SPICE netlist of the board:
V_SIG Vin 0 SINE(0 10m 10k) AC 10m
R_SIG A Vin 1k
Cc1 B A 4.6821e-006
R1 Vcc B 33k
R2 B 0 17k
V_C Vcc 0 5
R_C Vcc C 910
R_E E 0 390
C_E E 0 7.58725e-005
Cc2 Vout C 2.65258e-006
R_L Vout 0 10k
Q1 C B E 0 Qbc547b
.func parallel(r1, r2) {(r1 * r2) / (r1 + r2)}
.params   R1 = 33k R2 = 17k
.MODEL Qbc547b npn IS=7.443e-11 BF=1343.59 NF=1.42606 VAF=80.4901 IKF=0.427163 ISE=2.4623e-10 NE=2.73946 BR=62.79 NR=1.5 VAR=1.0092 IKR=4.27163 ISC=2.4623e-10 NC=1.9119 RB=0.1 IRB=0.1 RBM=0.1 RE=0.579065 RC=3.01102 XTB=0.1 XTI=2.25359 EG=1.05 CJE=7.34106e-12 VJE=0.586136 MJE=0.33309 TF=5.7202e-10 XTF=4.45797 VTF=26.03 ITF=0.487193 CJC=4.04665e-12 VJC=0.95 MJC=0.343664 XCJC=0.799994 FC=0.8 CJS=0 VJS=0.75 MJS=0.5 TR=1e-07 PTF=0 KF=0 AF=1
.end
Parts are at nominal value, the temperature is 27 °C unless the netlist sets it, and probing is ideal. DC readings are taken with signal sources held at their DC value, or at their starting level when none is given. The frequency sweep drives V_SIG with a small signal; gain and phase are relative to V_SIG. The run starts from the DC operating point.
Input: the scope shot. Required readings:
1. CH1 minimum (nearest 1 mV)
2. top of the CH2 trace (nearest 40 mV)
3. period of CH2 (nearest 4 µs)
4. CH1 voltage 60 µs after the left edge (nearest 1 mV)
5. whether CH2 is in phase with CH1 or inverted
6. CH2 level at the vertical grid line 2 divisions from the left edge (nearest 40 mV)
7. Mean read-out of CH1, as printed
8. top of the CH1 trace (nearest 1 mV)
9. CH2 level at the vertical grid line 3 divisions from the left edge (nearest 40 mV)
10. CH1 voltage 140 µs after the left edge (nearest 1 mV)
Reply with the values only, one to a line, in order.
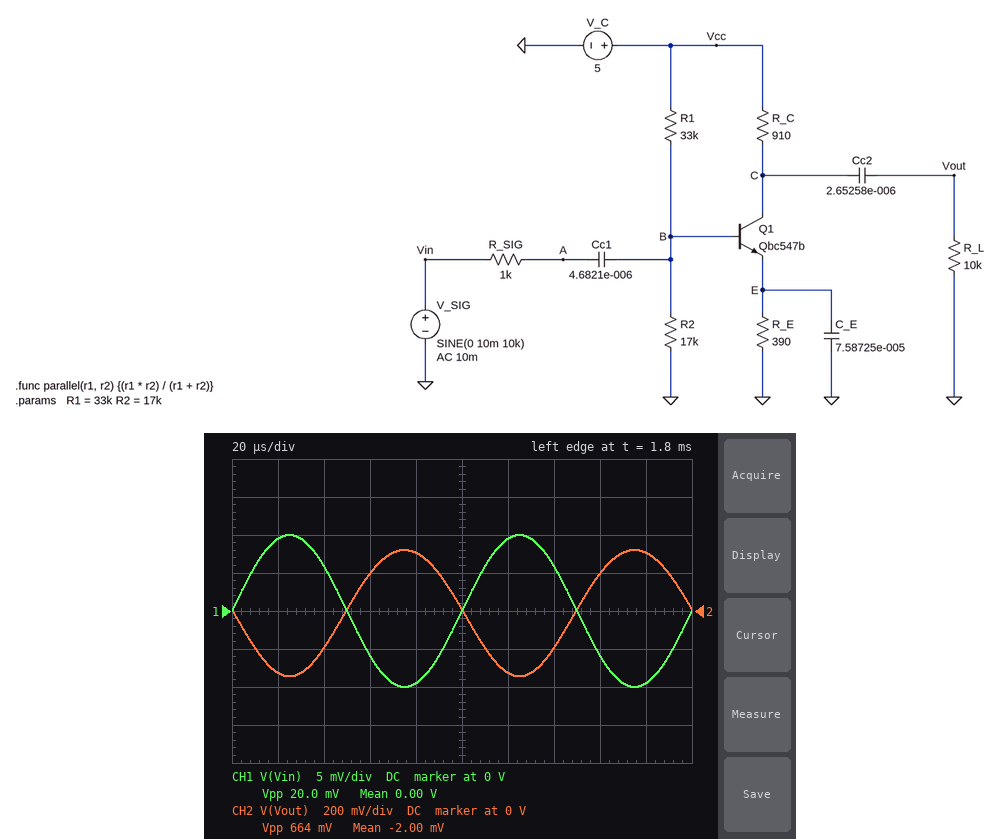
-10 mV
320 mV
100 µs
-6 mV
inverted
-200 mV
0.00 V
10 mV
200 mV
6 mV
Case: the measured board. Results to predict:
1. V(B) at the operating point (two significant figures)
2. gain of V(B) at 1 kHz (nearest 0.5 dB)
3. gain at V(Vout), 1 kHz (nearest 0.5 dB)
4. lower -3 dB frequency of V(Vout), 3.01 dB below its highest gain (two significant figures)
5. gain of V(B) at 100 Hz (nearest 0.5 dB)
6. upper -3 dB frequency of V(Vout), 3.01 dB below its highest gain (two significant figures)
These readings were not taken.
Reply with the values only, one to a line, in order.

1.6 V
-2.0 dB
30.5 dB
100 Hz
-1.5 dB
1.1 MHz
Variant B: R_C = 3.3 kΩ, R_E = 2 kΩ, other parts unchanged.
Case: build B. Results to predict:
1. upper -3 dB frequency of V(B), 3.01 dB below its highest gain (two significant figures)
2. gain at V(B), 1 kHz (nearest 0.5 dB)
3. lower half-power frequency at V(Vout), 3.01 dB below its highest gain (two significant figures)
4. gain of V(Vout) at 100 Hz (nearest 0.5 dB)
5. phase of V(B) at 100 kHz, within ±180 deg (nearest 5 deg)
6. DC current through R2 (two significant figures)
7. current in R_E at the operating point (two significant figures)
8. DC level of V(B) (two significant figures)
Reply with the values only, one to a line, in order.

1.5 MHz
-1.0 dB
28 Hz
28.5 dB
-5 deg
98 µA
530 µA
1.7 V
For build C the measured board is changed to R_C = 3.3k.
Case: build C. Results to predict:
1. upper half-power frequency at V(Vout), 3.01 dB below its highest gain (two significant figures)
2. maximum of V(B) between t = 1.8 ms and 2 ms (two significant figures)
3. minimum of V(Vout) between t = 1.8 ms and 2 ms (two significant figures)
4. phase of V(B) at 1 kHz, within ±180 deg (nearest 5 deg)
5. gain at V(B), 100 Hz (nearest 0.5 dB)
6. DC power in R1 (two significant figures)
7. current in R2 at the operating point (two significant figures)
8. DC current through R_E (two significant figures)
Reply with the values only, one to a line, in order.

200 kHz
1.2 V
-8.6 mV
0 deg
-19.5 dB
440 µW
70 µA
1.4 mA
